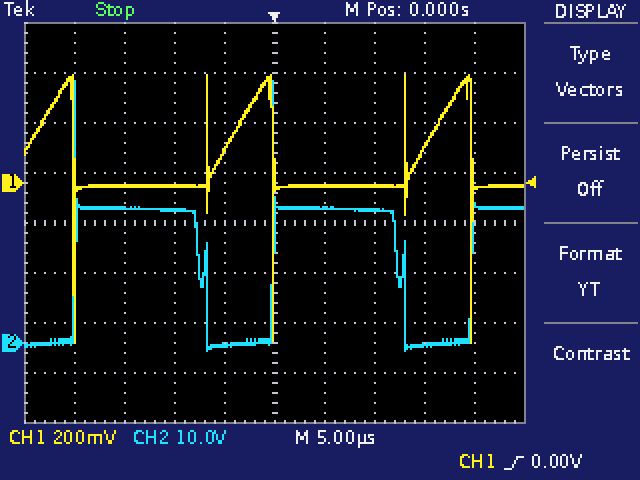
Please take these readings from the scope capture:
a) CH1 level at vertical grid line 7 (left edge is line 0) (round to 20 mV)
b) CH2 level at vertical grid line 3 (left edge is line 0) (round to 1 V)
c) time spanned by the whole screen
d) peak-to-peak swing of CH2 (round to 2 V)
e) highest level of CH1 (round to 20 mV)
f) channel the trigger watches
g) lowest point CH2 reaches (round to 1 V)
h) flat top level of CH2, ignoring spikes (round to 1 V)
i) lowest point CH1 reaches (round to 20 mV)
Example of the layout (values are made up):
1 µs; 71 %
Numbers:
-20 mV; 27 V; 50 µs; 54 V; 440 mV; CH1; -2 V; 27 V; -640 mV
